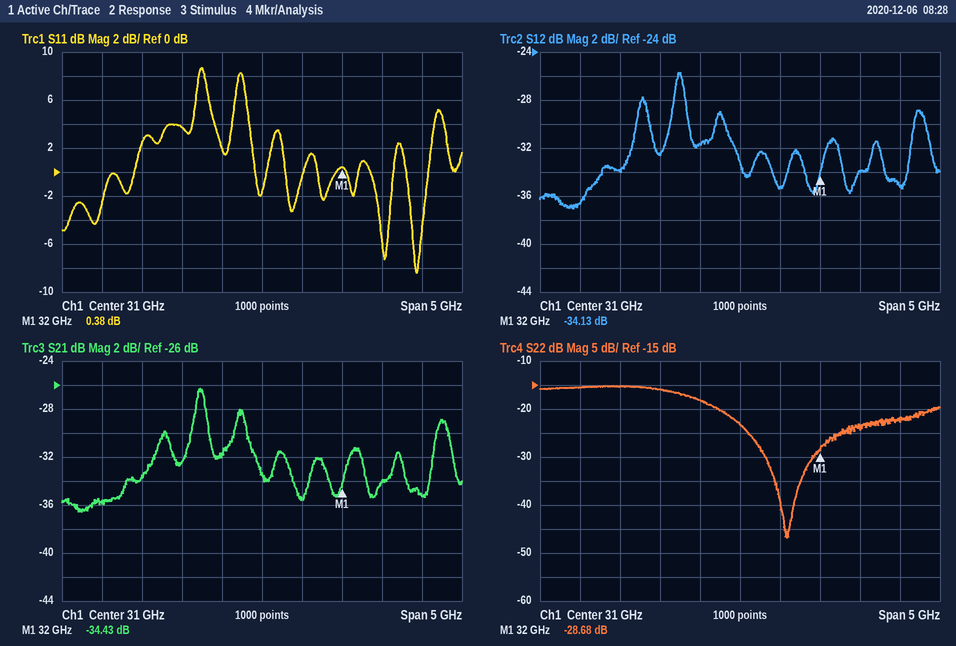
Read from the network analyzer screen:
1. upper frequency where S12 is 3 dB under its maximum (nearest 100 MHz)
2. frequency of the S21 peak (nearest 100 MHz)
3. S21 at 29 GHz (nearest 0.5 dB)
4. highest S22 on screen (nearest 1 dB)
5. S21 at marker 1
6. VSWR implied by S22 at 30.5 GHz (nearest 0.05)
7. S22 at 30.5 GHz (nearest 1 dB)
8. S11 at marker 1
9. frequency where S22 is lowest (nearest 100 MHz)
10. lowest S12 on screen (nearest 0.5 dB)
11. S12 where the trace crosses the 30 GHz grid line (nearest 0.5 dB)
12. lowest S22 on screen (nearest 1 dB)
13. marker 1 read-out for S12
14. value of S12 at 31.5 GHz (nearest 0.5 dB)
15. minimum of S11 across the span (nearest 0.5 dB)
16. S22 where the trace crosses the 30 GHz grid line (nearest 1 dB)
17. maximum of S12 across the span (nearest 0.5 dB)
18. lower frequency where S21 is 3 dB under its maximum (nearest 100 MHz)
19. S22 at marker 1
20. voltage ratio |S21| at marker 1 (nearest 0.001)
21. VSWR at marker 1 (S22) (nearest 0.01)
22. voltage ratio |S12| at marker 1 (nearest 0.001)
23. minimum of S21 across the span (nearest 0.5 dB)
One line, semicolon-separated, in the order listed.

30.3 GHz; 30.2 GHz; -36.0 dB; -15 dB; -34.43 dB; 1.30; -18 dB; 0.38 dB; 31.6 GHz; -37.0 dB; -32.5 dB; -47 dB; -34.13 dB; -35.5 dB; -8.5 dB; -16 dB; -25.5 dB; 30.1 GHz; -28.68 dB; 0.019; 1.08; 0.020; -36.5 dB
